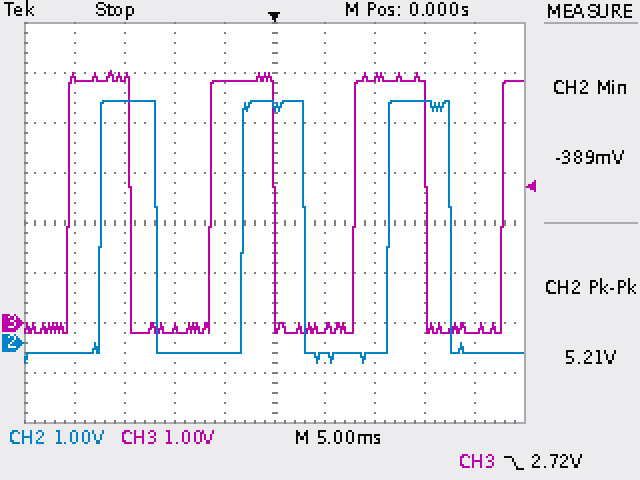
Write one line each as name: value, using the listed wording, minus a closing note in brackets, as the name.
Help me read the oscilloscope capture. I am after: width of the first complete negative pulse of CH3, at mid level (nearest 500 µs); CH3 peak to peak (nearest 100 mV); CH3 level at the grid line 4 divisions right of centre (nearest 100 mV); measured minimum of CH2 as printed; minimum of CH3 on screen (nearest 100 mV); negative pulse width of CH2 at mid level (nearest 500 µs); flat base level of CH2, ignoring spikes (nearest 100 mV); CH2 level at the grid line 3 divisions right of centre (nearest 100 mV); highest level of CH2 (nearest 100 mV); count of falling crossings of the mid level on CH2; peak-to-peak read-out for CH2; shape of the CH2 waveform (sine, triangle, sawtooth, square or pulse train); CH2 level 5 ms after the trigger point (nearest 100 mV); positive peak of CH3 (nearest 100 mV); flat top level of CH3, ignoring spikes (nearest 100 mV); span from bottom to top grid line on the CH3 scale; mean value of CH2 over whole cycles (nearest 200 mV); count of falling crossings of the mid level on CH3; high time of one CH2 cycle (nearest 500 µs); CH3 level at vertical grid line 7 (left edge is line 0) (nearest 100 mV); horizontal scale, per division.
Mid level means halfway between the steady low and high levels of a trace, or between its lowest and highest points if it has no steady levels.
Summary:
width of the first complete negative pulse of CH3, at mid level: 8.0 ms
CH3 peak to peak: 5.2 V
CH3 level at the grid line 4 divisions right of centre: -200 mV
measured minimum of CH2 as printed: -389 mV
minimum of CH3 on screen: -200 mV
negative pulse width of CH2 at mid level: 8.5 ms
flat base level of CH2, ignoring spikes: -200 mV
CH2 level at the grid line 3 divisions right of centre: 4.8 V
highest level of CH2: 4.8 V
count of falling crossings of the mid level on CH2: 3
peak-to-peak read-out for CH2: 5.21 V
shape of the CH2 waveform: pulse train
CH2 level 5 ms after the trigger point: -200 mV
positive peak of CH3: 5.0 V
flat top level of CH3, ignoring spikes: 4.8 V
span from bottom to top grid line on the CH3 scale: 8 V
mean value of CH2 over whole cycles: 1.8 V
count of falling crossings of the mid level on CH3: 3
high time of one CH2 cycle: 6.0 ms
CH3 level at vertical grid line 7 (left edge is line 0): 4.9 V
horizontal scale, per division: 5 ms
